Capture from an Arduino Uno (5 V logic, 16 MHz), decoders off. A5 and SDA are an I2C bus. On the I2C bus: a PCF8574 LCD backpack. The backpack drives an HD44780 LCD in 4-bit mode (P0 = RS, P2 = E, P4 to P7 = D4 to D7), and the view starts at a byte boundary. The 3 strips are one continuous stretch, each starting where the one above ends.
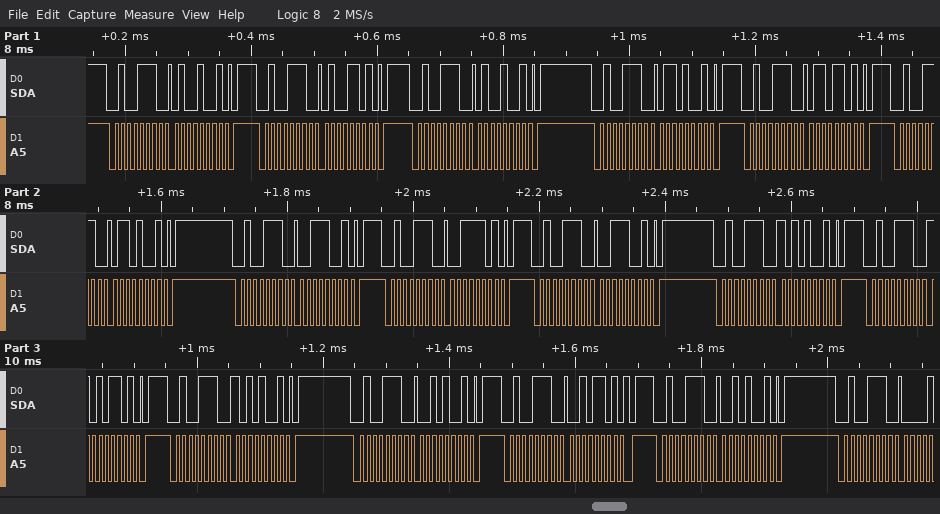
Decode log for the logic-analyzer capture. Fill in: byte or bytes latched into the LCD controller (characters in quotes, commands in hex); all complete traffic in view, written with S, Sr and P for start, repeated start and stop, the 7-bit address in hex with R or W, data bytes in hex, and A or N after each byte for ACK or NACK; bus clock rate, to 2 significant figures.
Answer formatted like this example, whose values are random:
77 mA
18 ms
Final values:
'F' ':'
S 27W A 49 A P S 27W A 4D A P S 27W A 49 A P S 27W A 69 A P S 27W A 6D A P S 27W A 69 A P S 27W A 39 A P S 27W A 3D A P S 27W A 39 A P S 27W A A9 A P S 27W A AD A P S 27W A A9 A P S 27W A 29 A P S 27W A 2D A P S 27W A 29 A P S 27W A
100 kHz
